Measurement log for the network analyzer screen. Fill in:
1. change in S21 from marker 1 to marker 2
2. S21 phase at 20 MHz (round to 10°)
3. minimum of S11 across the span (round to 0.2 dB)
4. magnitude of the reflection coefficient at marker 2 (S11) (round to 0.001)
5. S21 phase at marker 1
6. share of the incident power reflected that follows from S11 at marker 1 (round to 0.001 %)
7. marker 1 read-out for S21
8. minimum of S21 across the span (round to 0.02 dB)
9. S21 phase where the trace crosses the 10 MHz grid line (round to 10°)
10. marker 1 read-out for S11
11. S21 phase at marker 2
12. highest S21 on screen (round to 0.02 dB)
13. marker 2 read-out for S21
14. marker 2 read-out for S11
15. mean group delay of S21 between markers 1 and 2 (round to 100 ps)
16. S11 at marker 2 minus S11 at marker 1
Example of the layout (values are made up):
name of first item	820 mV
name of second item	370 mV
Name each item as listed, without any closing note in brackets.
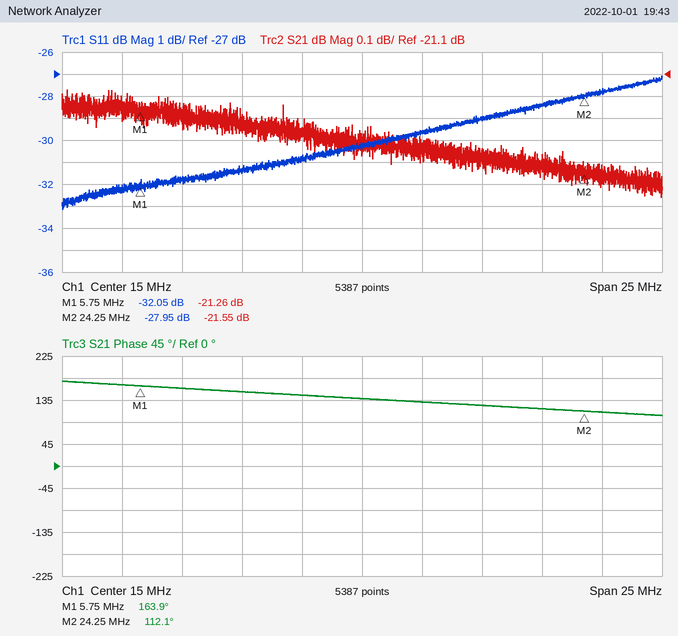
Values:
change in S21 from marker 1 to marker 2	-0.29 dB
S21 phase at 20 MHz	120°
minimum of S11 across the span	-33.2 dB
magnitude of the reflection coefficient at marker 2 (S11)	0.040
S21 phase at marker 1	163.9°
share of the incident power reflected that follows from S11 at marker 1	0.062 %
marker 1 read-out for S21	-21.26 dB
minimum of S21 across the span	-21.66 dB
S21 phase where the trace crosses the 10 MHz grid line	150°
marker 1 read-out for S11	-32.05 dB
S21 phase at marker 2	112.1°
highest S21 on screen	-21.18 dB
marker 2 read-out for S21	-21.55 dB
marker 2 read-out for S11	-27.95 dB
mean group delay of S21 between markers 1 and 2	7.8 ns
S11 at marker 2 minus S11 at marker 1	4.10 dB
